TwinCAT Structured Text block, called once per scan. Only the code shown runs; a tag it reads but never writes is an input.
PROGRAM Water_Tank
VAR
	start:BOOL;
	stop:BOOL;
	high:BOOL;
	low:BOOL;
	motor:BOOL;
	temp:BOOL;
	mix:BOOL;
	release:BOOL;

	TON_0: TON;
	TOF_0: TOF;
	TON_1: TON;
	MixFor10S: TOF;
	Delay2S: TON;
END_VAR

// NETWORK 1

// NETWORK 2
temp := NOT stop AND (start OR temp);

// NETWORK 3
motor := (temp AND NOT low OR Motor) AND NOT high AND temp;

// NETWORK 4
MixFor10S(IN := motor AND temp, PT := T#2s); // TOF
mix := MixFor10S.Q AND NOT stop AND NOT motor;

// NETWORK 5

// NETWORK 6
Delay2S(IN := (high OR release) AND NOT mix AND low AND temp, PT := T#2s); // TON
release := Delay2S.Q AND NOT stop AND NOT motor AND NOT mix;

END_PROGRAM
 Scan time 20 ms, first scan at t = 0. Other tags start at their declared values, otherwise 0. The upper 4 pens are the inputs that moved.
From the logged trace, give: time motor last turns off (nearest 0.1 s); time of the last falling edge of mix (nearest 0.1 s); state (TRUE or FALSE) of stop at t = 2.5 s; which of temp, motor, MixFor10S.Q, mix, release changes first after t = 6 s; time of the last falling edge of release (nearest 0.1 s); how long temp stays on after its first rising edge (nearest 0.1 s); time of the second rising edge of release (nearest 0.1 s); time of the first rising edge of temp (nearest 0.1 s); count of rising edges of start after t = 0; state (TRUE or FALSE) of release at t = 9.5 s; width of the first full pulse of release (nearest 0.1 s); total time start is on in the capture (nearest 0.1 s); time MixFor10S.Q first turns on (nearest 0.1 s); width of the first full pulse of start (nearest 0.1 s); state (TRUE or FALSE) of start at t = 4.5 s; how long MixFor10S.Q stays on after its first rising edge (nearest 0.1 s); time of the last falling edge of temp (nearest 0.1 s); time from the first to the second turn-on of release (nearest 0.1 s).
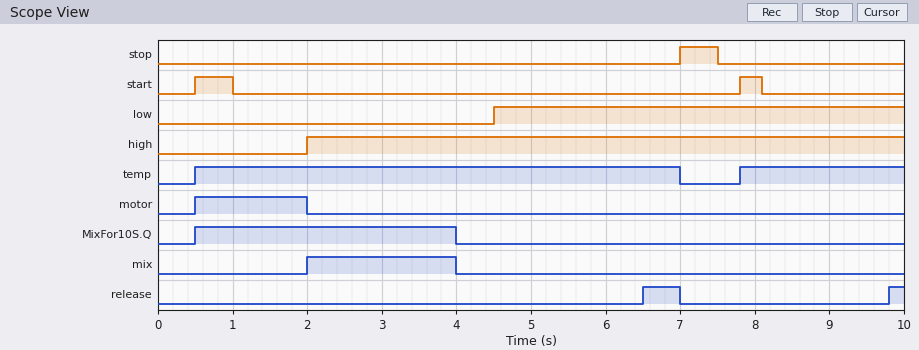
2.0 s
4.0 s
FALSE
release
7.0 s
6.5 s
9.8 s
0.5 s
2
FALSE
0.5 s
0.8 s
0.5 s
0.5 s
FALSE
3.5 s
7.0 s
3.3 s
